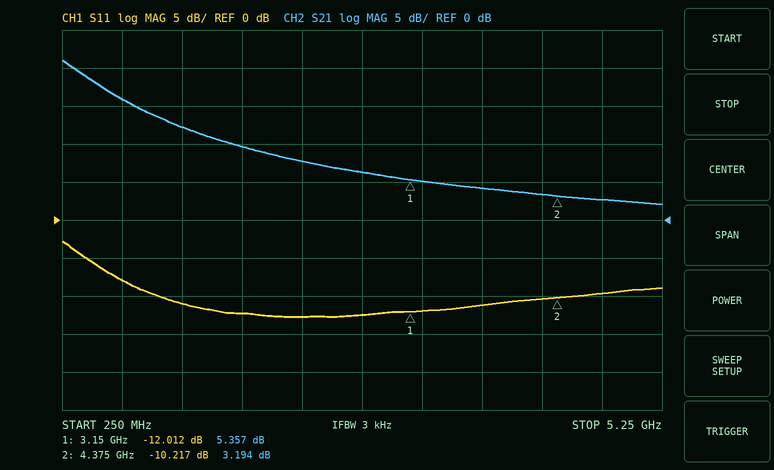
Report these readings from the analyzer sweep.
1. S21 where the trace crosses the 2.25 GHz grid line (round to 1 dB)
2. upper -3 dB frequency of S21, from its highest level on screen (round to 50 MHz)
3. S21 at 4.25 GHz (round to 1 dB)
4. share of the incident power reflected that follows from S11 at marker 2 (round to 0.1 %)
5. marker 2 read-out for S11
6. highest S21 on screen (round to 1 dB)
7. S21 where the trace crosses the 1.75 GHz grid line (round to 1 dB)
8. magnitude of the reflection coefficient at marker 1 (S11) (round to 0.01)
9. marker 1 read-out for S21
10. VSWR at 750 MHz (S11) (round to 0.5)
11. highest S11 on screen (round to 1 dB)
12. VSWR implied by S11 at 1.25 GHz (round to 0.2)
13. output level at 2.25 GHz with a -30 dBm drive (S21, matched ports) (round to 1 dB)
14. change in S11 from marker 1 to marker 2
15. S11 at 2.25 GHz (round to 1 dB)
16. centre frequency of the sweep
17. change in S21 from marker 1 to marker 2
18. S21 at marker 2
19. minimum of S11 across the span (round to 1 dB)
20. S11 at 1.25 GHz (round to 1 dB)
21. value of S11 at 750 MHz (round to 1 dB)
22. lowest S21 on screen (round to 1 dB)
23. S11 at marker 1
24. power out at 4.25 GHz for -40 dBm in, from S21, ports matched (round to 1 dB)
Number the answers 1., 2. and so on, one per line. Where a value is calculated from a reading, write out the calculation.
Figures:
1. 8 dB
2. 550 MHz
3. 3 dB
4. 10^(-10.217/10) ≈ 9.5 %
5. -10.217 dB
6. 21 dB
7. 10 dB
8. 10^(-12.012/20) ≈ 0.25
9. 5.357 dB
10. |Γ| = 10^(-8/20) = 0.3981; VSWR = (1 + 0.3981)/(1 − 0.3981) ≈ 2.32, so 2.5 to the nearest 0.5
11. -3 dB
12. |Γ| = 10^(-11/20) = 0.2818; VSWR = (1 + 0.2818)/(1 − 0.2818) ≈ 1.8
13. -30 dBm + (8 dB) = -22 dBm
14. -10.217 − (-12.012) = 1.795 dB
15. -13 dB
16. 2.75 GHz
17. 3.194 − (5.357) = -2.163 dB
18. 3.194 dB
19. -13 dB
20. -11 dB
21. -8 dB
22. 2 dB
23. -12.012 dB
24. -40 dBm + (3 dB) = -37 dBm
